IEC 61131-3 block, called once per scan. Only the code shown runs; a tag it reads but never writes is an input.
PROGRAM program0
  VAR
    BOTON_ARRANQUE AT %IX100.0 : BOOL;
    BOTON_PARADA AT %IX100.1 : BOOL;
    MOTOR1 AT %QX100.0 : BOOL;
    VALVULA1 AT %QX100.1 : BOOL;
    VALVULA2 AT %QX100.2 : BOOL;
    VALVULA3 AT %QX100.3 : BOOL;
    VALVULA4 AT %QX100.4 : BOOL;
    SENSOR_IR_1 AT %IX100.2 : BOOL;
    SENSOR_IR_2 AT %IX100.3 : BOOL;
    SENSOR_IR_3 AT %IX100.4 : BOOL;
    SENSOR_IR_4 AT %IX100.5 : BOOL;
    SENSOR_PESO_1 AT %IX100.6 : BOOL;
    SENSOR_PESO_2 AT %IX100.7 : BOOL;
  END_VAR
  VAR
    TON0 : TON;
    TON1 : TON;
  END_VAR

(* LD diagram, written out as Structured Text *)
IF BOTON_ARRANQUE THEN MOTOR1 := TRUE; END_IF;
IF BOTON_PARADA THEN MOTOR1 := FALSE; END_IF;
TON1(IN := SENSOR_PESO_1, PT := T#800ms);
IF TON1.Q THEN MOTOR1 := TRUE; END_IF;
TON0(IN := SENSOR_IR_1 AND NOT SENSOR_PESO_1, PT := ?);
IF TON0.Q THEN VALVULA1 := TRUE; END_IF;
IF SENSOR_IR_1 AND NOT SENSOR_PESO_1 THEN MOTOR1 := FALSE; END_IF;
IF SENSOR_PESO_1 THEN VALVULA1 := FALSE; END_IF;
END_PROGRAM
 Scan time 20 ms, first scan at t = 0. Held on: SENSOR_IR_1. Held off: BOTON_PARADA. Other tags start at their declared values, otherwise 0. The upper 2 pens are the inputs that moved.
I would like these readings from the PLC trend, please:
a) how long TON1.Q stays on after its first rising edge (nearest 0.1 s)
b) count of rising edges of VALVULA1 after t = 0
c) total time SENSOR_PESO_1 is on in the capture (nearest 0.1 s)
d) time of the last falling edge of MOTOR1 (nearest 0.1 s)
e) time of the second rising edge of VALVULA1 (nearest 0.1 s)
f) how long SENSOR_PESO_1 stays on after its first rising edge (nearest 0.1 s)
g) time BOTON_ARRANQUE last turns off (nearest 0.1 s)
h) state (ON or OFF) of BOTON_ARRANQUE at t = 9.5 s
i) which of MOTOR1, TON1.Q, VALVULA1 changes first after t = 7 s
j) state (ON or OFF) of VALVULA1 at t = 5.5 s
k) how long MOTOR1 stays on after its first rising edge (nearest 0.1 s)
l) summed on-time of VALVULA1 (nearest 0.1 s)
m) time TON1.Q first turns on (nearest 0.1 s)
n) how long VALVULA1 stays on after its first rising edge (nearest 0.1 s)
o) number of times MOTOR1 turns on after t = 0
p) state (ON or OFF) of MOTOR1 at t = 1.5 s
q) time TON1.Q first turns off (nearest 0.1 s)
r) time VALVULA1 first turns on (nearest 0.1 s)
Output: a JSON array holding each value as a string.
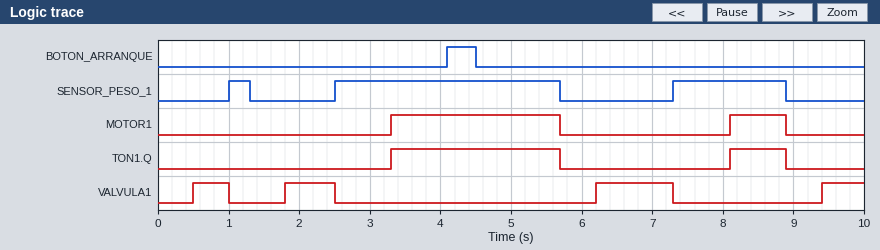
["2.4 s", "4", "5.1 s", "8.9 s", "1.8 s", "0.3 s", "4.5 s", "OFF", "VALVULA1", "OFF", "2.4 s", "2.9 s", "3.3 s", "0.5 s", "2", "OFF", "5.7 s", "0.5 s"]
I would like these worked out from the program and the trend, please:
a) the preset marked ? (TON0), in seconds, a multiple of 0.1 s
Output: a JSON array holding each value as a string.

["0.5 s"]
